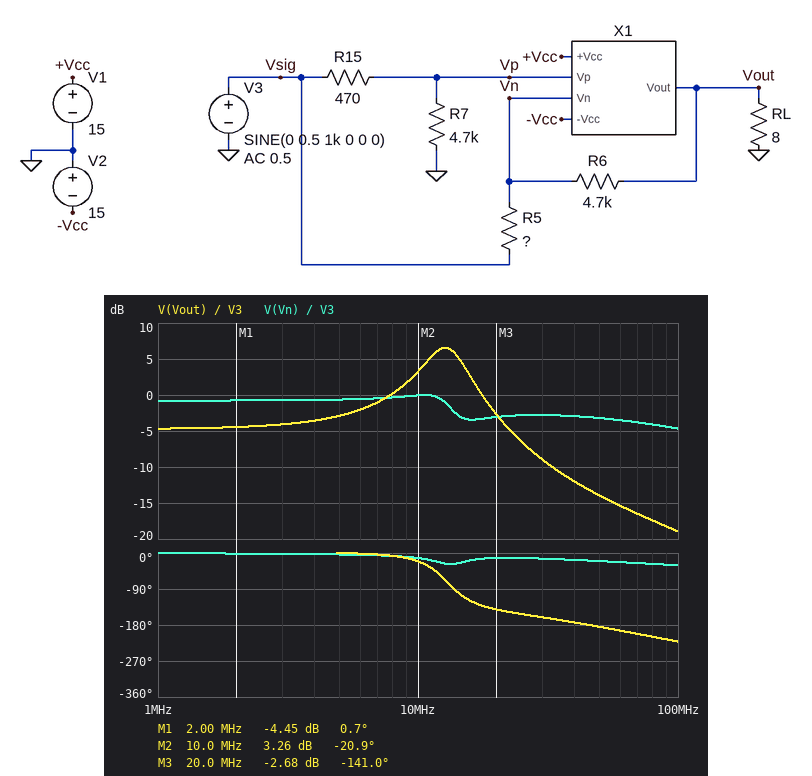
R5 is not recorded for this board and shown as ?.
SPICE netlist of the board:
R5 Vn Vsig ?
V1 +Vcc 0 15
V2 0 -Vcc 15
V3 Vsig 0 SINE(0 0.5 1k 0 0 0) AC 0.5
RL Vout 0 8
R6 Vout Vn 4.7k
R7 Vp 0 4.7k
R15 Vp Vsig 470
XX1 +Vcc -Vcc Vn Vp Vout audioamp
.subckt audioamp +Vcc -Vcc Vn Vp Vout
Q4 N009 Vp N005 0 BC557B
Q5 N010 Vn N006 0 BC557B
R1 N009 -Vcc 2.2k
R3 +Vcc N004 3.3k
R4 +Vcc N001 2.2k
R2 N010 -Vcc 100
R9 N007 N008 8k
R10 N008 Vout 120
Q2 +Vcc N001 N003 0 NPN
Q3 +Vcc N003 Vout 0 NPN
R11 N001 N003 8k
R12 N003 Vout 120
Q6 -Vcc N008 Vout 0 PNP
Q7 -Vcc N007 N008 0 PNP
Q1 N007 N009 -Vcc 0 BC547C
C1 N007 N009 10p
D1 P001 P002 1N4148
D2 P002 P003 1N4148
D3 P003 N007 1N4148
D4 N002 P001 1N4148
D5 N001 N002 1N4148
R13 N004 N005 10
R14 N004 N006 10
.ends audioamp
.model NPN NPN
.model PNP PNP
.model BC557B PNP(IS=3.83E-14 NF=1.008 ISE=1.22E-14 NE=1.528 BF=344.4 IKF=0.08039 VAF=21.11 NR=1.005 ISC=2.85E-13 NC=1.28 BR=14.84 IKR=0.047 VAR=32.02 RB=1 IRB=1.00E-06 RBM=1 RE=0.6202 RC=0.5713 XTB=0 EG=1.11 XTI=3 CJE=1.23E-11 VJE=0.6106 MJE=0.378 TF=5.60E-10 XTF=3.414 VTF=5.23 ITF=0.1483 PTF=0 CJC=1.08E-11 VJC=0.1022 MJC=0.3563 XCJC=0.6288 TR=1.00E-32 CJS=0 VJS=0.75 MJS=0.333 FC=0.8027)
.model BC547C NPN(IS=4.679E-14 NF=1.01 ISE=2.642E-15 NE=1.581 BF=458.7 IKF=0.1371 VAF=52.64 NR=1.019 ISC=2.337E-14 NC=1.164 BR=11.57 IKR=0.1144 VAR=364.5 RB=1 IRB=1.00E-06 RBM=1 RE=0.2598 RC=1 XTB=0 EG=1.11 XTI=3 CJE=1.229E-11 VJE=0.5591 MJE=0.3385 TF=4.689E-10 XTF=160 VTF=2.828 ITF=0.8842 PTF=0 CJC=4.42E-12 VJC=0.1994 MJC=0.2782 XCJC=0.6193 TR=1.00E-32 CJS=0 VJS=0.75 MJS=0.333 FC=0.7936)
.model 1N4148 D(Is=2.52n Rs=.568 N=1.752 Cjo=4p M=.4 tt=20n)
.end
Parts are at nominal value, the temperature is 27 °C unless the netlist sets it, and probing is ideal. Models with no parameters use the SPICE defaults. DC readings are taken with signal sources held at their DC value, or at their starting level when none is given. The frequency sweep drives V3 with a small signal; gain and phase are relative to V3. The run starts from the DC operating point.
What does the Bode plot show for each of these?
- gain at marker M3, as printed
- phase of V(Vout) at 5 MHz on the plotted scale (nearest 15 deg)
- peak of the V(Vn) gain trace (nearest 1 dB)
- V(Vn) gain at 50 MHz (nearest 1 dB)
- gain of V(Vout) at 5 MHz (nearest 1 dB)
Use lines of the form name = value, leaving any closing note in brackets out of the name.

gain at marker M3, as printed = -2.68 dB
phase of V(Vout) at 5 MHz on the plotted scale = 0 deg
peak of the V(Vn) gain trace = 0 dB
V(Vn) gain at 50 MHz = -3 dB
gain of V(Vout) at 5 MHz = -3 dB
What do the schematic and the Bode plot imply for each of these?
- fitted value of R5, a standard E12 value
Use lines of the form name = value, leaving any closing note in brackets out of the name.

fitted value of R5, a standard E12 value = 1.2 kΩ
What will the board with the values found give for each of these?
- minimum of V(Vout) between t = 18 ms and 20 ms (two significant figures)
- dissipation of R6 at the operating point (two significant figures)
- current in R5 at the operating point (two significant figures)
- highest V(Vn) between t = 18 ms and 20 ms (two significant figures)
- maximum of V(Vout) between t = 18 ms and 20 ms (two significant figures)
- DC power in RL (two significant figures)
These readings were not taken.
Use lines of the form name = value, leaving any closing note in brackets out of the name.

minimum of V(Vout) between t = 18 ms and 20 ms = -850 mV
dissipation of R6 at the operating point = 44 µW
current in R5 at the operating point = 89 µA
highest V(Vn) between t = 18 ms and 20 ms = 350 mV
maximum of V(Vout) between t = 18 ms and 20 ms = -270 mV
DC power in RL = 39 mW
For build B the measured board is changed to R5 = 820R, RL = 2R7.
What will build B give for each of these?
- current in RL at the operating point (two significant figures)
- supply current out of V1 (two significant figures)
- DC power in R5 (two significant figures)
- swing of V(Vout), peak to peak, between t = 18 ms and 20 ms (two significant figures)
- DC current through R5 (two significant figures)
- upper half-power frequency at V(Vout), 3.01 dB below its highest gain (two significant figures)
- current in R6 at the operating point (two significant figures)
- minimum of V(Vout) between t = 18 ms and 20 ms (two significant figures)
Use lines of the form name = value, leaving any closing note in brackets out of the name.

current in RL at the operating point = 280 mA
supply current out of V1 = 18 mA
DC power in R5 = 14 µW
swing of V(Vout), peak to peak, between t = 18 ms and 20 ms = 420 mV
DC current through R5 = 130 µA
upper half-power frequency at V(Vout), 3.01 dB below its highest gain = 15 MHz
current in R6 at the operating point = 140 µA
minimum of V(Vout) between t = 18 ms and 20 ms = -960 mV
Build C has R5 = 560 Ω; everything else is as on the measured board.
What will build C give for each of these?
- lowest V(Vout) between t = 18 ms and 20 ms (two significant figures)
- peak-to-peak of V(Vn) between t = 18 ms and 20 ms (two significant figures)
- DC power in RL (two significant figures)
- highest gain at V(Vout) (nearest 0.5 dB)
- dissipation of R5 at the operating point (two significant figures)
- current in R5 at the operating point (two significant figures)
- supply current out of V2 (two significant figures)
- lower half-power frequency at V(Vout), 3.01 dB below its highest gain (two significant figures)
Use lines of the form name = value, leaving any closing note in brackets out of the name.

lowest V(Vout) between t = 18 ms and 20 ms = -1.1 V
peak-to-peak of V(Vn) between t = 18 ms and 20 ms = 910 mV
DC power in RL = 130 mW
highest gain at V(Vout) = -7.0 dB
dissipation of R5 at the operating point = 20 µW
current in R5 at the operating point = 190 µA
supply current out of V2 = 150 mA
lower half-power frequency at V(Vout), 3.01 dB below its highest gain = 6.5 MHz
